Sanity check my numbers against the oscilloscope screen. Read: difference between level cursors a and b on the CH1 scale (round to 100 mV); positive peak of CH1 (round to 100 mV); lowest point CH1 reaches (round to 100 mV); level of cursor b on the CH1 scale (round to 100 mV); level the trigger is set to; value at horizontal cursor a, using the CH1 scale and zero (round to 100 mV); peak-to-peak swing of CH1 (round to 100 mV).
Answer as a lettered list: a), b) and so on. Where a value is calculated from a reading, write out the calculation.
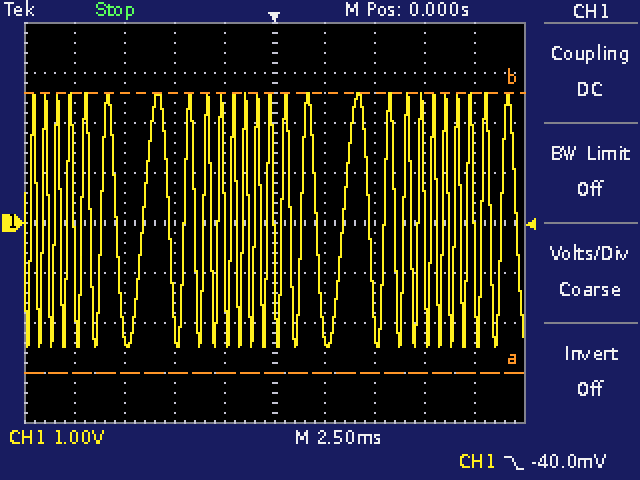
a) 5.6 V
b) 2.6 V
c) -2.5 V
d) 2.6 V
e) -40.0 mV
f) -3.0 V
g) 2.6 V − (-2.5 V) = 5.1 V
